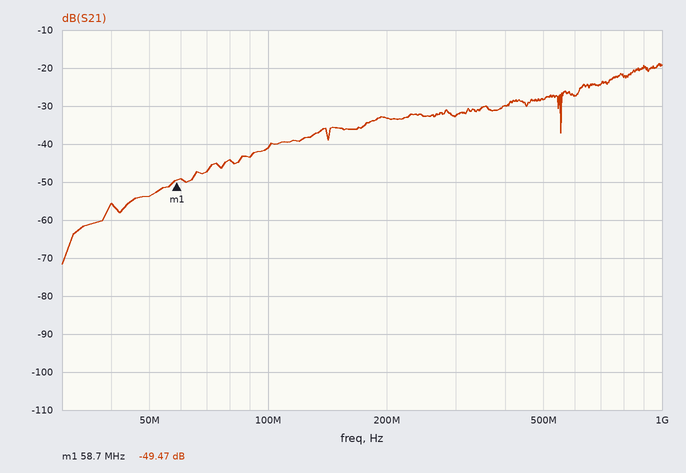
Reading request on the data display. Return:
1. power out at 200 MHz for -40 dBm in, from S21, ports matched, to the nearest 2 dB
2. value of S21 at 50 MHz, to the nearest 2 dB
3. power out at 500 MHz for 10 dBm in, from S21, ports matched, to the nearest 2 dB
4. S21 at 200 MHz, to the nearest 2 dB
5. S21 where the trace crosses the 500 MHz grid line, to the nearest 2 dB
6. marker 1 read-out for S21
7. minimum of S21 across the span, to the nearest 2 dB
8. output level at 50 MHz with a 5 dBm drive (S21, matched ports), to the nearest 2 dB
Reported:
-74 dBm
-54 dB
-18 dBm
-34 dB
-28 dB
-49.47 dB
-72 dB
-48 dBm
